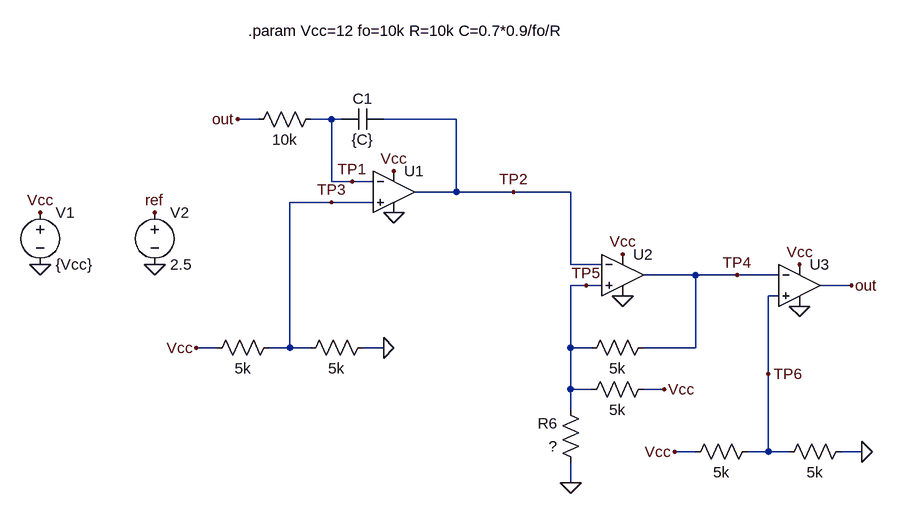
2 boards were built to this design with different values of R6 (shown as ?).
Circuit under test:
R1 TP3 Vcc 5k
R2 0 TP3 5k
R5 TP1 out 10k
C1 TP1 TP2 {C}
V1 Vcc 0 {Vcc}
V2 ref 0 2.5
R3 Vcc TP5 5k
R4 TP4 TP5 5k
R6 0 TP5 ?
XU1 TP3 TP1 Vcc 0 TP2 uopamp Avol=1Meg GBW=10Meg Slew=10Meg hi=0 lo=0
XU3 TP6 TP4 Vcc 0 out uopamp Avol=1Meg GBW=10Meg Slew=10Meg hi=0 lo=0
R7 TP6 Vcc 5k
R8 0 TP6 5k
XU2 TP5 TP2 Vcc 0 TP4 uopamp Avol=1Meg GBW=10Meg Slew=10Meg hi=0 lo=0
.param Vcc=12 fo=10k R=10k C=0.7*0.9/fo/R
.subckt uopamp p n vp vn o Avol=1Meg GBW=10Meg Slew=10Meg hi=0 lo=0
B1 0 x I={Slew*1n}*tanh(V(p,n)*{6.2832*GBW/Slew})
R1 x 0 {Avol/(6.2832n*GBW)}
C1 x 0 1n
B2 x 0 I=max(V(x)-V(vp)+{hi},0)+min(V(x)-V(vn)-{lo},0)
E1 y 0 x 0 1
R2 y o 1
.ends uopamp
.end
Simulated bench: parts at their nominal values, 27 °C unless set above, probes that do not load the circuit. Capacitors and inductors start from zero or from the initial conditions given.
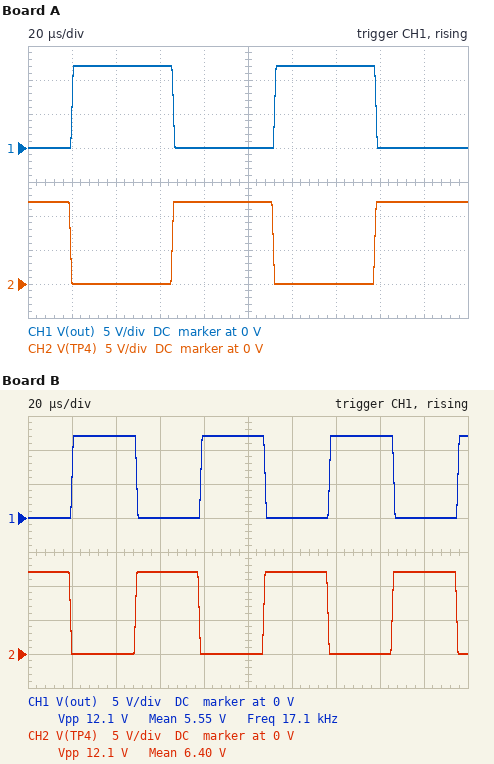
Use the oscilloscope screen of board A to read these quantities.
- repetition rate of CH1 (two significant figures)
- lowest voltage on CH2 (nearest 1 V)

11 kHz
0 V
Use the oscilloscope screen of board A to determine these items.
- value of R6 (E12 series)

5.6 kΩ
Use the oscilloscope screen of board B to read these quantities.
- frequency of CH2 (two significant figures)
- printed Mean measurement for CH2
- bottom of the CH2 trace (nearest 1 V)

17 kHz
6.40 V
0 V
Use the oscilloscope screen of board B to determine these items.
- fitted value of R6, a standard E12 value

1.8 kΩ
